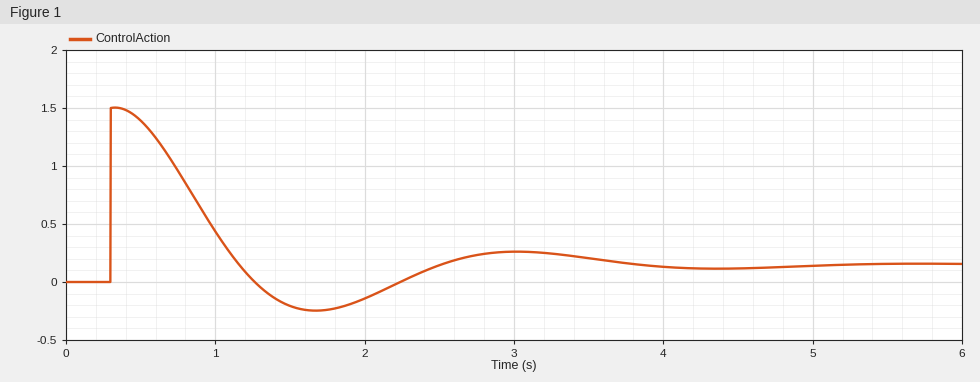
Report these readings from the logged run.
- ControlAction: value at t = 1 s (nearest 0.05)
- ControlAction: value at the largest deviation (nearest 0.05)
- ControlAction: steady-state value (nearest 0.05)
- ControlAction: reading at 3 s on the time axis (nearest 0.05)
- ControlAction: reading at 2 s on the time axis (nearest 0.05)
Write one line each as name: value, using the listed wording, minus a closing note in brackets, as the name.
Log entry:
ControlAction: value at t = 1 s: 0.45
ControlAction: value at the largest deviation: 1.50
ControlAction: steady-state value: 0.15
ControlAction: reading at 3 s on the time axis: 0.25
ControlAction: reading at 2 s on the time axis: -0.15
